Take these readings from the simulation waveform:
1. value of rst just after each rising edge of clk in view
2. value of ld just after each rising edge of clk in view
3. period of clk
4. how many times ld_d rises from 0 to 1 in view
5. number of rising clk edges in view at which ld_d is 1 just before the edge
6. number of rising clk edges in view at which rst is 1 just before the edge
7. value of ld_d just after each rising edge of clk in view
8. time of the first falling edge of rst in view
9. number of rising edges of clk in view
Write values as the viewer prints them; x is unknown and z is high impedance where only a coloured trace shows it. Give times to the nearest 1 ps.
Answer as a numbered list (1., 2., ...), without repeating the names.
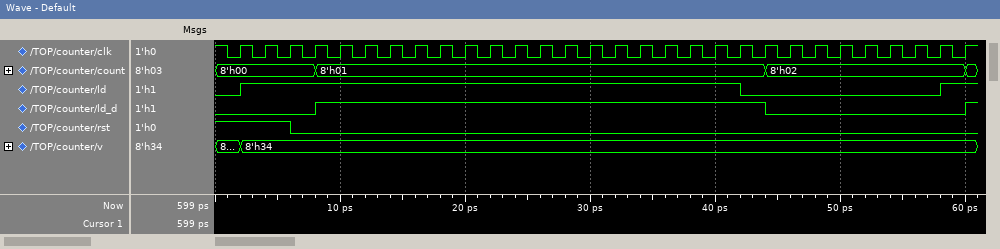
1. 1 1 0 0 0 0 0 0 0 0 0 0 0 0 0 0 0 0 0 0 0 0 0 0 0 0 0 0 0 0
2. 1 1 1 1 1 1 1 1 1 1 1 1 1 1 1 1 1 1 1 1 0 0 0 0 0 0 0 0 1 1
3. 2 ps
4. 2
5. 18
6. 3
7. 0 0 0 1 1 1 1 1 1 1 1 1 1 1 1 1 1 1 1 1 1 0 0 0 0 0 0 0 0 1
8. 6 ps
9. 30
